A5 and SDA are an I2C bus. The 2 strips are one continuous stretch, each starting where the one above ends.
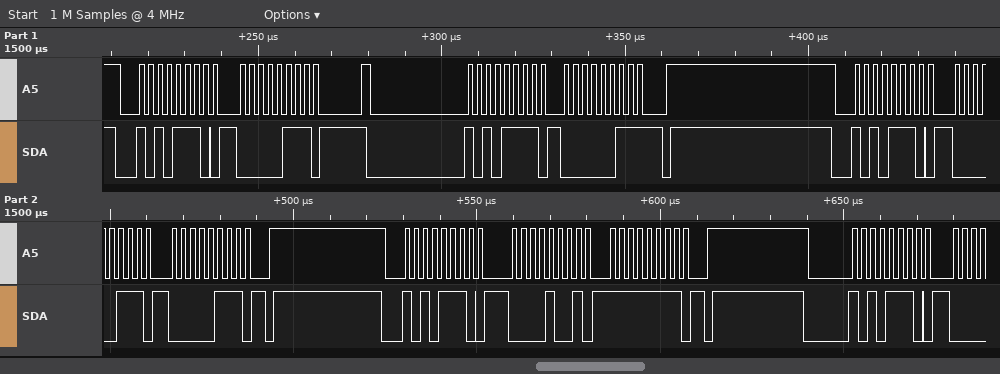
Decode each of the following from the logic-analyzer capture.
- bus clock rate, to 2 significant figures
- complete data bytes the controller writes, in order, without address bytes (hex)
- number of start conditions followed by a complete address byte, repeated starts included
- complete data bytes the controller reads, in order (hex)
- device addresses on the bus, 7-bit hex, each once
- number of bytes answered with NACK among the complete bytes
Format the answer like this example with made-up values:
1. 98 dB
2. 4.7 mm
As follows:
1. 400 kHz
2. 07 07 07 09 FF
3. 5
4. 03
5. 0x57
6. 1
